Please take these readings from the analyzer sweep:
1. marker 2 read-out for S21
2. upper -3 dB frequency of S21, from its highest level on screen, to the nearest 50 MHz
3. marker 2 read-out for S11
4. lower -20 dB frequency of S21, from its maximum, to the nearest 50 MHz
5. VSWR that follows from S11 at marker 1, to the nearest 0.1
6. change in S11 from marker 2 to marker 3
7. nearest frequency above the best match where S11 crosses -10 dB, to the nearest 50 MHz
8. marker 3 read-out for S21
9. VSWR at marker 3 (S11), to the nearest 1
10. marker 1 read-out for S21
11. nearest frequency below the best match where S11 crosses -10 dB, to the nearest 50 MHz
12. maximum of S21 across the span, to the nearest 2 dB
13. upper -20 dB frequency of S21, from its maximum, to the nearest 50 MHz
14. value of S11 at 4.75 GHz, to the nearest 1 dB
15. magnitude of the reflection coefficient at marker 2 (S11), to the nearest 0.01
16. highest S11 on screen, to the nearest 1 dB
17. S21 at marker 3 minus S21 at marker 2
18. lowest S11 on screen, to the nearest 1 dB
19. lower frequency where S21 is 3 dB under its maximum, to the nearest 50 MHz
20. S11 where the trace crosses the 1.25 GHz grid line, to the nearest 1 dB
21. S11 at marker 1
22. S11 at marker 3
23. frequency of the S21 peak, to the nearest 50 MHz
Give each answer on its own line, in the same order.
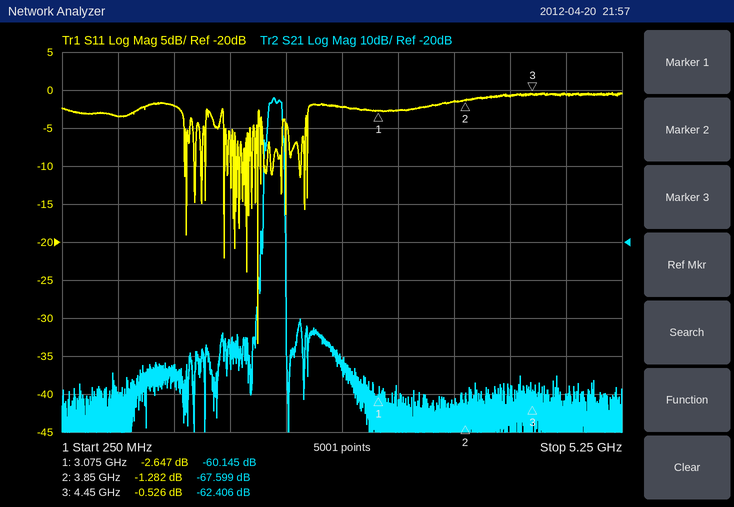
-67.599 dB
2.20 GHz
-1.282 dB
2.05 GHz
6.6
0.756 dB
2.00 GHz
-62.406 dB
33
-60.145 dB
2.00 GHz
18 dB
2.25 GHz
-1 dB
0.86
0 dB
5.193 dB
-33 dB
2.10 GHz
-2 dB
-2.647 dB
-0.526 dB
2.15 GHz
